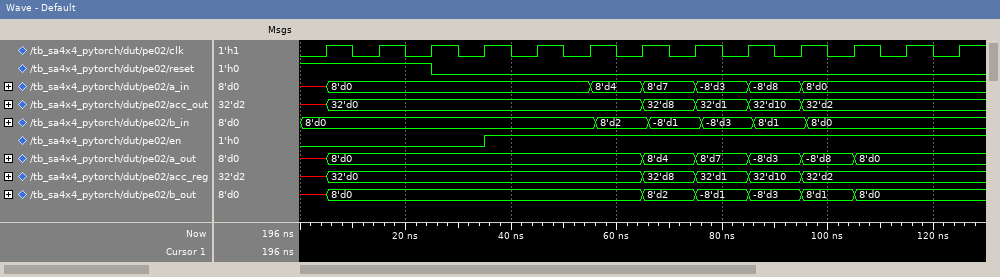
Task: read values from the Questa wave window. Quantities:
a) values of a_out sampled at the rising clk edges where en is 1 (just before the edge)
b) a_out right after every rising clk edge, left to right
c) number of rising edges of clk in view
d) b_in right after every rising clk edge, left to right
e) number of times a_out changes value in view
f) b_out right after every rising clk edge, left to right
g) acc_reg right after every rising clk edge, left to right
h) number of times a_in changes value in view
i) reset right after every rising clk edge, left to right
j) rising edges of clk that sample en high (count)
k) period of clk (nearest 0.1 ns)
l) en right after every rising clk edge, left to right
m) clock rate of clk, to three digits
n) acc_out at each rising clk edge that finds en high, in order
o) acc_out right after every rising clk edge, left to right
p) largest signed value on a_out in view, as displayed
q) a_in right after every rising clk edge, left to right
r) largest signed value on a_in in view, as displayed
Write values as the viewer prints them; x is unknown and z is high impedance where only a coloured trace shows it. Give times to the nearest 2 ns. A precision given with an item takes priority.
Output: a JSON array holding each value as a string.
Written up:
["8'd0, 8'd0, 8'd0, 8'd4, 8'd7, -8'd3, -8'd8, 8'd0, 8'd0", "8'd0, 8'd0, 8'd0, 8'd0, 8'd0, 8'd0, 8'd4, 8'd7, -8'd3, -8'd8, 8'd0, 8'd0, 8'd0", "13", "8'd0, 8'd0, 8'd0, 8'd0, 8'd0, 8'd0, 8'd2, -8'd1, -8'd3, 8'd1, 8'd0, 8'd0, 8'd0", "6", "8'd0, 8'd0, 8'd0, 8'd0, 8'd0, 8'd0, 8'd2, -8'd1, -8'd3, 8'd1, 8'd0, 8'd0, 8'd0", "32'd0, 32'd0, 32'd0, 32'd0, 32'd0, 32'd0, 32'd8, 32'd1, 32'd10, 32'd2, 32'd2, 32'd2, 32'd2", "6", "1 1 0 0 0 0 0 0 0 0 0 0 0", "9", "10 ns", "0 0 0 1 1 1 1 1 1 1 1 1 1", "100 MHz", "32'd0, 32'd0, 32'd0, 32'd8, 32'd1, 32'd10, 32'd2, 32'd2, 32'd2", "32'd0, 32'd0, 32'd0, 32'd0, 32'd0, 32'd0, 32'd8, 32'd1, 32'd10, 32'd2, 32'd2, 32'd2, 32'd2", "8'd7", "8'd0, 8'd0, 8'd0, 8'd0, 8'd0, 8'd4, 8'd7, -8'd3, -8'd8, 8'd0, 8'd0, 8'd0, 8'd0", "8'd7"]
